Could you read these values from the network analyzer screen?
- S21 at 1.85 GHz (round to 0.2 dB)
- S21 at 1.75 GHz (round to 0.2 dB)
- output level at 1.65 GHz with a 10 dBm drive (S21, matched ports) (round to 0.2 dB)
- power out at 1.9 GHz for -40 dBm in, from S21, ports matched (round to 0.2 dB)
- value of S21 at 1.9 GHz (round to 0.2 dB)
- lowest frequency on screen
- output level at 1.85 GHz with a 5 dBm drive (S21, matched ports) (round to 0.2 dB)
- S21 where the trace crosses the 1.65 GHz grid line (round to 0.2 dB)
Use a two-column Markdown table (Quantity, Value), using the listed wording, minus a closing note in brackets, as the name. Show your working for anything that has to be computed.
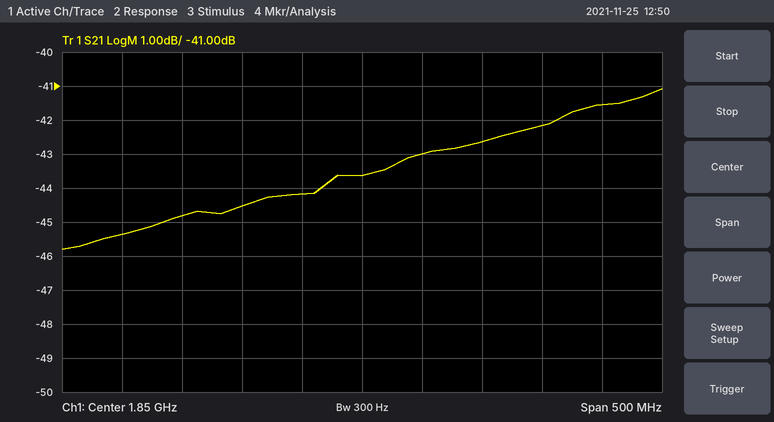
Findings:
| Quantity | Value |
|---|---|
| S21 at 1.85 GHz | -43.6 dB |
| S21 at 1.75 GHz | -44.6 dB |
| output level at 1.65 GHz with a 10 dBm drive (S21, matched ports) | 10 dBm + (-45.4 dB) = -35.4 dBm |
| power out at 1.9 GHz for -40 dBm in, from S21, ports matched | -40 dBm + (-43.0 dB) = -83.0 dBm |
| value of S21 at 1.9 GHz | -43.0 dB |
| lowest frequency on screen | 1.6 GHz |
| output level at 1.85 GHz with a 5 dBm drive (S21, matched ports) | 5 dBm + (-43.6 dB) = -38.6 dBm |
| S21 where the trace crosses the 1.65 GHz grid line | -45.4 dB |
